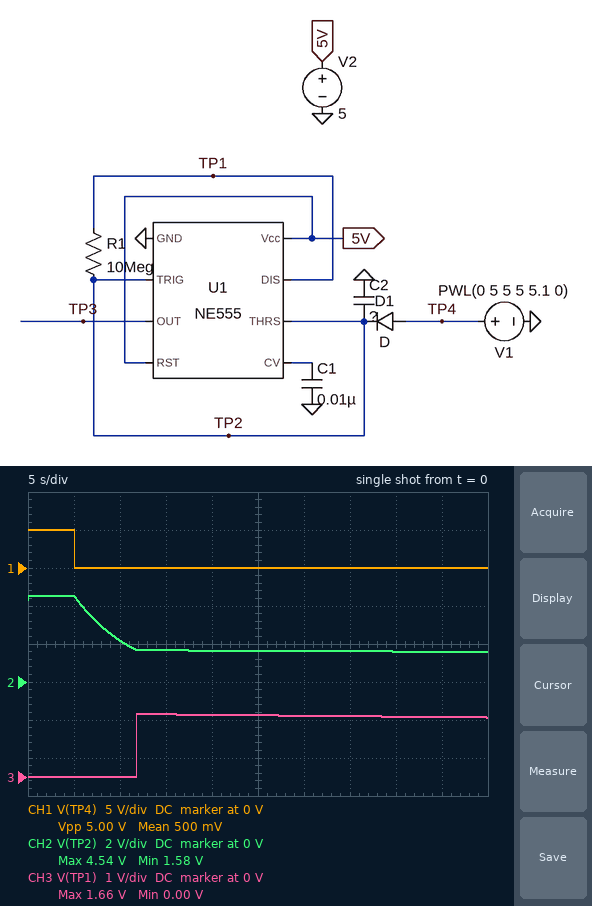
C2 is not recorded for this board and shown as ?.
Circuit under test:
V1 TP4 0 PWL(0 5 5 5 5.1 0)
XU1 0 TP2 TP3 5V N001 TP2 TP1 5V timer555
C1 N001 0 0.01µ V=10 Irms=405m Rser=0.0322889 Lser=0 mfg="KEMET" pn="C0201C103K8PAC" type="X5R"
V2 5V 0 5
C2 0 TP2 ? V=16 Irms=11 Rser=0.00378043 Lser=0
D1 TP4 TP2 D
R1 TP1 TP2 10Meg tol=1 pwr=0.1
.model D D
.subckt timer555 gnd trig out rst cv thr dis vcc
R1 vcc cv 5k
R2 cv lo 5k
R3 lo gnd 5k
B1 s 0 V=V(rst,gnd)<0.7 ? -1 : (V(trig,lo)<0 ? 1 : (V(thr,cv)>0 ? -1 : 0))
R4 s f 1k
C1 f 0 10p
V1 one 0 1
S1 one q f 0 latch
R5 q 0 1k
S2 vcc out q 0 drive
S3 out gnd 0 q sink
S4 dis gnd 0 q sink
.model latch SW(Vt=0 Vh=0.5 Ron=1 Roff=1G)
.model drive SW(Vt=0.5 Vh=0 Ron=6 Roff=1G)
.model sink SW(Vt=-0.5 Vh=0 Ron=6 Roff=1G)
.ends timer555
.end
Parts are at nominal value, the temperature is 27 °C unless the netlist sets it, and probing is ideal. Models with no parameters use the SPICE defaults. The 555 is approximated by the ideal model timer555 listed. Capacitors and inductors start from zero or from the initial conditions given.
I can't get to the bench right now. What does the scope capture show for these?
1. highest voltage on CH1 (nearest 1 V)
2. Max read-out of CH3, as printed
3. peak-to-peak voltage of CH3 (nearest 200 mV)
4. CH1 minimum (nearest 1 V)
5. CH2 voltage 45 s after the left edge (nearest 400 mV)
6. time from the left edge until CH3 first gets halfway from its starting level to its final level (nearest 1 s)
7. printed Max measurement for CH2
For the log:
5 V
1.66 V
1.6 V
0 V
1.6 V
12 s
4.54 V
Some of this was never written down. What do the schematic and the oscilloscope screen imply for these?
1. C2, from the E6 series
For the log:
680 nF
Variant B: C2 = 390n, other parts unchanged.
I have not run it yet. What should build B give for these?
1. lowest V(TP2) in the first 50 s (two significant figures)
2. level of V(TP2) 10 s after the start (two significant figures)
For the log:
1.5 V
1.7 V
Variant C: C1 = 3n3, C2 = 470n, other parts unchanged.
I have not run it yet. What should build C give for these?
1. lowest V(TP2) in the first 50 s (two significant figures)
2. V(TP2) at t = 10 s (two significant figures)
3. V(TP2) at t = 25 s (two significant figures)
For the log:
1.5 V
1.7 V
1.6 V
